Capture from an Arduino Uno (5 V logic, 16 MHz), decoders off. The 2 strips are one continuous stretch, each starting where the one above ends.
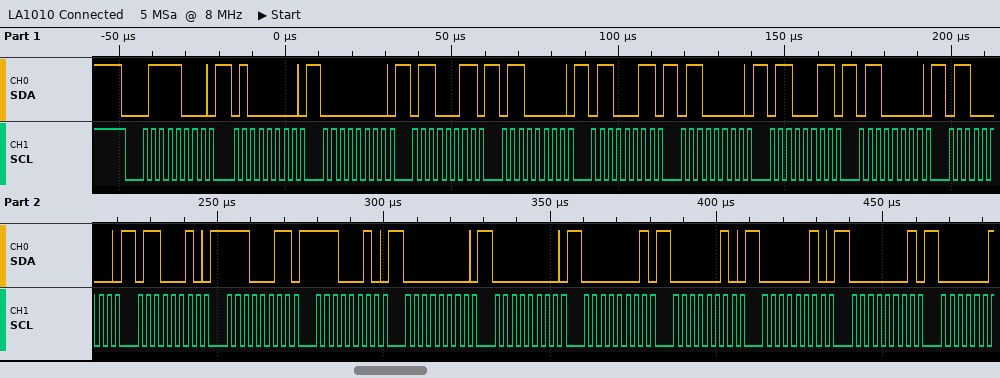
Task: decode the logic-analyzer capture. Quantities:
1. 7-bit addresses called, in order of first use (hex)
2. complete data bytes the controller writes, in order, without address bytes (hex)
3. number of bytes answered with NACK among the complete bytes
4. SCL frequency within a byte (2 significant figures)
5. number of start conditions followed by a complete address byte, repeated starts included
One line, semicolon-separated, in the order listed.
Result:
0x3C; 40 00 63 60 63 60 63 60 60 62 E3 E2 00 00 01 02 02 01; 0; 400 kHz; 1
